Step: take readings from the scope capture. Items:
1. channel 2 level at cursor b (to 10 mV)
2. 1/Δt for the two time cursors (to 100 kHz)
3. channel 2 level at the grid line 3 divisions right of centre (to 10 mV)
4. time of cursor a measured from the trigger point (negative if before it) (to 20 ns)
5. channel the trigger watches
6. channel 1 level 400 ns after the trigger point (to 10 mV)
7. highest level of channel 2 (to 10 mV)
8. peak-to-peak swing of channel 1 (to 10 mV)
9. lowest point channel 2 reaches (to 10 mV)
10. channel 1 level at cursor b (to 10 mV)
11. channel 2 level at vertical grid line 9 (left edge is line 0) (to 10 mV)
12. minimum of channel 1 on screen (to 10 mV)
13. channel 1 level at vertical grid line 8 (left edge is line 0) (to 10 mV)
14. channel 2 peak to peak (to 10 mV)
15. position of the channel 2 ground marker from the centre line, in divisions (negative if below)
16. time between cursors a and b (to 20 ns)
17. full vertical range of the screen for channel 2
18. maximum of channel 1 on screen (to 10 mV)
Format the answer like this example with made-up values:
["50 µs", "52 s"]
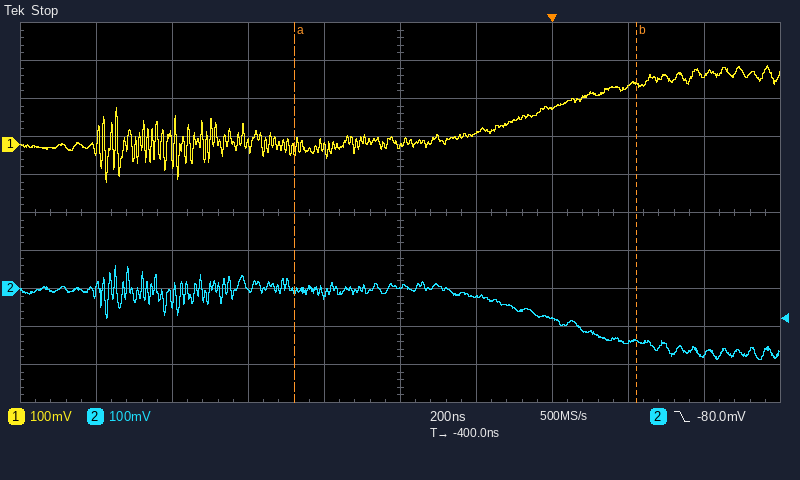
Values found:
["-140 mV", "1.1 MHz", "-140 mV", "-680 ns", "channel 2", "180 mV", "60 mV", "310 mV", "-190 mV", "160 mV", "-170 mV", "-100 mV", "150 mV", "250 mV", "-2.0 div", "900 ns", "1 V", "210 mV"]
